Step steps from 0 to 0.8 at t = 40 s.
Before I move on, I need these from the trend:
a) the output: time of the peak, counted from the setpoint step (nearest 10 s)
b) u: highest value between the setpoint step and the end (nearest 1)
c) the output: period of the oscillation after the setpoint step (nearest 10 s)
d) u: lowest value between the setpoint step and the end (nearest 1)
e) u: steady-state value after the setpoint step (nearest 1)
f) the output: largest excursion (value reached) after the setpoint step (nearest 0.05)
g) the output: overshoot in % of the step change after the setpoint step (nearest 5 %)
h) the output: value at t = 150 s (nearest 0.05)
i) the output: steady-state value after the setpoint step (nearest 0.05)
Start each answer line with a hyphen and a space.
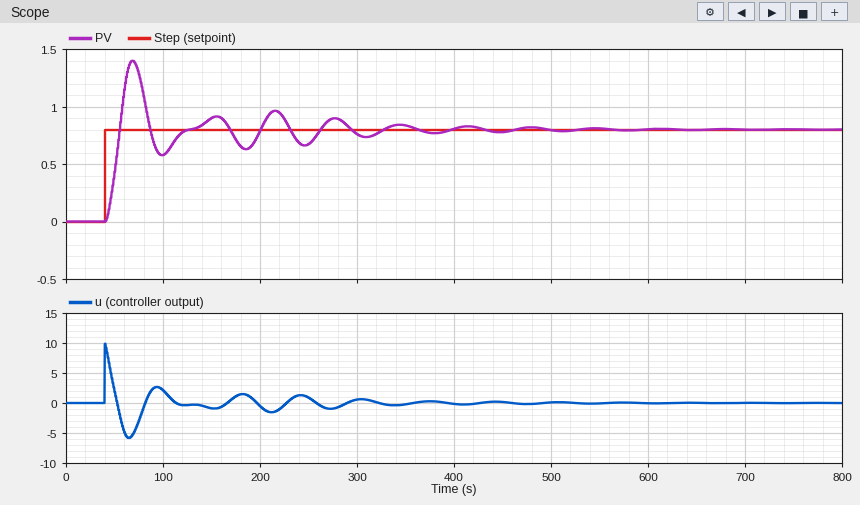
- 30 s
- 10
- 90 s
- -6
- 0
- 1.40
- 75 %
- 0.90
- 0.80
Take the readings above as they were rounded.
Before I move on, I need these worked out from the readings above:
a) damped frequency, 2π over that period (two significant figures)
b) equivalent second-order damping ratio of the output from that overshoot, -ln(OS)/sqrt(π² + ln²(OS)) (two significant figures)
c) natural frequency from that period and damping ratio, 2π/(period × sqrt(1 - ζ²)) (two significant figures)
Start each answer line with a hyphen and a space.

- 0.070 rad/s
- 0.091
- 0.070 rad/s
